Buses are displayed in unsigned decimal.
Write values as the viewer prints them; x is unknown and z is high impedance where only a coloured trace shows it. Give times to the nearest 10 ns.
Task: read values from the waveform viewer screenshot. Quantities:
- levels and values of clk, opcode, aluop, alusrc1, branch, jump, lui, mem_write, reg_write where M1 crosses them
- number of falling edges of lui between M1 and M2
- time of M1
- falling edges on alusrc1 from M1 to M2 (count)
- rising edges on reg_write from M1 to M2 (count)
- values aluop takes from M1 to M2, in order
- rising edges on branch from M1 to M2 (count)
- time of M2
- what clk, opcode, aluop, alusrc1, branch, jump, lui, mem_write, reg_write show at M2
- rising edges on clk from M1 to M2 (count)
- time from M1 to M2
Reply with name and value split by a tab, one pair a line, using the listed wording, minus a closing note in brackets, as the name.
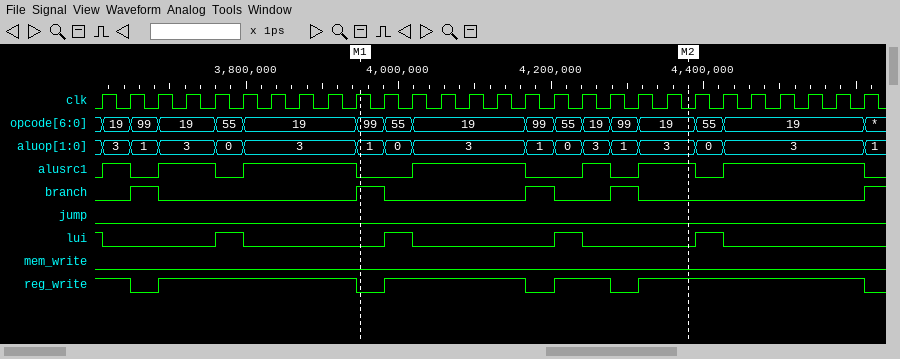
levels and values of clk, opcode, aluop, alusrc1, branch, jump, lui, mem_write, reg_write where M1 crosses them	clk=1, opcode=99, aluop=1, alusrc1=0, branch=1, jump=0, lui=0, mem_write=0, reg_write=0
number of falling edges of lui between M1 and M2	2
time of M1	3950 ns
falling edges on alusrc1 from M1 to M2	2
rising edges on reg_write from M1 to M2	3
values aluop takes from M1 to M2, in order	1, 0, 3, 1, 0, 3, 1, 3
rising edges on branch from M1 to M2	2
time of M2	4380 ns
what clk, opcode, aluop, alusrc1, branch, jump, lui, mem_write, reg_write show at M2	clk=0, opcode=19, aluop=3, alusrc1=1, branch=0, jump=0, lui=0, mem_write=0, reg_write=1
rising edges on clk from M1 to M2	11
time from M1 to M2	430 ns
